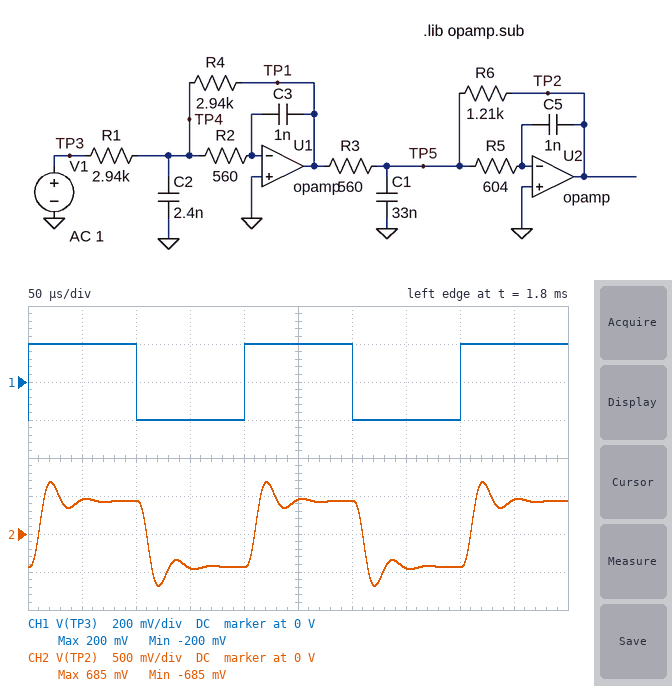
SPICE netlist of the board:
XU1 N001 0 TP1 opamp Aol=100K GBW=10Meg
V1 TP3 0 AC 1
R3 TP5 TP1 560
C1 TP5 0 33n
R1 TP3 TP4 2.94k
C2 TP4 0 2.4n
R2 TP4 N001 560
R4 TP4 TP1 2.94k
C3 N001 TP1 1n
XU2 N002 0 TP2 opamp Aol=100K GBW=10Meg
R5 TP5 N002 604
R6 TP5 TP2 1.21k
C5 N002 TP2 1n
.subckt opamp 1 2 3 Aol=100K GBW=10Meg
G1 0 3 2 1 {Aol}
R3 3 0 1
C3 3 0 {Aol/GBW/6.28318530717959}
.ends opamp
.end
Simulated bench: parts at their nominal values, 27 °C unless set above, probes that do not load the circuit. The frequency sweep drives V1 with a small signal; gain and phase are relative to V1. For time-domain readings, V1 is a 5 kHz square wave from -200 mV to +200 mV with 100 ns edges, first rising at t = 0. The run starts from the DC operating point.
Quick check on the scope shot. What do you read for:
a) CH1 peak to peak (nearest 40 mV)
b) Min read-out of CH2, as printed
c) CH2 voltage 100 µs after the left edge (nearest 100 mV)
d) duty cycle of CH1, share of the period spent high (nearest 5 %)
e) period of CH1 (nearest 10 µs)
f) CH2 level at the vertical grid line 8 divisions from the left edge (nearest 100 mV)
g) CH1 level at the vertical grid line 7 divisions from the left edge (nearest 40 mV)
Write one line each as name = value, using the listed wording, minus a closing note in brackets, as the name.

CH1 peak to peak = 400 mV
Min read-out of CH2, as printed = -685 mV
CH2 voltage 100 µs after the left edge = 400 mV
duty cycle of CH1, share of the period spent high = 50 %
period of CH1 = 200 µs
CH2 level at the vertical grid line 8 divisions from the left edge = -400 mV
CH1 level at the vertical grid line 7 divisions from the left edge = -200 mV
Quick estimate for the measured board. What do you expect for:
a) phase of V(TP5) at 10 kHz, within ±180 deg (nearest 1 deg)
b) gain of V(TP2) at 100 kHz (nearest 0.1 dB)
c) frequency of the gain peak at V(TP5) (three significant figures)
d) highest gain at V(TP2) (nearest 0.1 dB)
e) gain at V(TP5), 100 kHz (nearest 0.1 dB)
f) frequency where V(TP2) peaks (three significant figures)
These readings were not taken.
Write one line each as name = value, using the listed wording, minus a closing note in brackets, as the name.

phase of V(TP5) at 10 kHz, within ±180 deg = -117 deg
gain of V(TP2) at 100 kHz = -20.8 dB
frequency of the gain peak at V(TP5) = 31.1 kHz
highest gain at V(TP2) = 10.0 dB
gain at V(TP5), 100 kHz = -29.0 dB
frequency where V(TP2) peaks = 27.6 kHz
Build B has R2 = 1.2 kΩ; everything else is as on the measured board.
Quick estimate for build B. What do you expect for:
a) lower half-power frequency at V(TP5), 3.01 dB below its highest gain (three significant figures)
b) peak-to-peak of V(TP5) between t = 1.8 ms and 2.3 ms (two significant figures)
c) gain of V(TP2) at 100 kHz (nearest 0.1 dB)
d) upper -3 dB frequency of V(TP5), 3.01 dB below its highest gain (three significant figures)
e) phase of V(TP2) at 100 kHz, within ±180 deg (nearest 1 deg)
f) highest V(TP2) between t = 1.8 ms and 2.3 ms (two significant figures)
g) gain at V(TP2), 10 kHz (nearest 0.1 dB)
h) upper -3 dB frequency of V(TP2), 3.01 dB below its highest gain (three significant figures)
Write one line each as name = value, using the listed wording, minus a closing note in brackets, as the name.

lower half-power frequency at V(TP5), 3.01 dB below its highest gain = 21.9 kHz
peak-to-peak of V(TP5) between t = 1.8 ms and 2.3 ms = 110 mV
gain of V(TP2) at 100 kHz = -24.7 dB
upper -3 dB frequency of V(TP5), 3.01 dB below its highest gain = 40.2 kHz
phase of V(TP2) at 100 kHz, within ±180 deg = 66 deg
highest V(TP2) between t = 1.8 ms and 2.3 ms = 660 mV
gain at V(TP2), 10 kHz = 7.2 dB
upper -3 dB frequency of V(TP2), 3.01 dB below its highest gain = 36.0 kHz
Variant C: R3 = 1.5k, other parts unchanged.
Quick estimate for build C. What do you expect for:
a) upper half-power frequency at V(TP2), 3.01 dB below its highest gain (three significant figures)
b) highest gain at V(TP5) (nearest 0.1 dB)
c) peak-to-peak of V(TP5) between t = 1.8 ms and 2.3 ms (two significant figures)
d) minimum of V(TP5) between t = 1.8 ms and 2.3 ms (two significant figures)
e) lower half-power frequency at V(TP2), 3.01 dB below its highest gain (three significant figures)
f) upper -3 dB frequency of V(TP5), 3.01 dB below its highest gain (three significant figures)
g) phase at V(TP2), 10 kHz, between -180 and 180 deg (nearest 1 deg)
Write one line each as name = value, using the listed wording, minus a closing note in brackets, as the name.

upper half-power frequency at V(TP2), 3.01 dB below its highest gain = 36.3 kHz
highest gain at V(TP5) = -14.7 dB
peak-to-peak of V(TP5) between t = 1.8 ms and 2.3 ms = 50 mV
minimum of V(TP5) between t = 1.8 ms and 2.3 ms = -25 mV
lower half-power frequency at V(TP2), 3.01 dB below its highest gain = 19.4 kHz
upper -3 dB frequency of V(TP5), 3.01 dB below its highest gain = 39.0 kHz
phase at V(TP2), 10 kHz, between -180 and 180 deg = -24 deg
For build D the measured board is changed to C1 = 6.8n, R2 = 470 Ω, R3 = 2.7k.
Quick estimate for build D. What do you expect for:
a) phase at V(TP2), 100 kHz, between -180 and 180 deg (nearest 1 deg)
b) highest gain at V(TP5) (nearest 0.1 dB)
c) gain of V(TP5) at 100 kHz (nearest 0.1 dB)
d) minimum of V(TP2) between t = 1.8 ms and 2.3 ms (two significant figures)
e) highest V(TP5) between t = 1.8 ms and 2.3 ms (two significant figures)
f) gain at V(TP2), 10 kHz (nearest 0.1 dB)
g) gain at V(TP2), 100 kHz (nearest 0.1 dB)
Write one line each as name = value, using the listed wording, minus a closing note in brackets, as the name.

phase at V(TP2), 100 kHz, between -180 and 180 deg = 133 deg
highest gain at V(TP5) = -21.9 dB
gain of V(TP5) at 100 kHz = -27.4 dB
minimum of V(TP2) between t = 1.8 ms and 2.3 ms = -100 mV
highest V(TP5) between t = 1.8 ms and 2.3 ms = 18 mV
gain at V(TP2), 10 kHz = -7.0 dB
gain at V(TP2), 100 kHz = -19.2 dB
